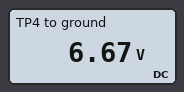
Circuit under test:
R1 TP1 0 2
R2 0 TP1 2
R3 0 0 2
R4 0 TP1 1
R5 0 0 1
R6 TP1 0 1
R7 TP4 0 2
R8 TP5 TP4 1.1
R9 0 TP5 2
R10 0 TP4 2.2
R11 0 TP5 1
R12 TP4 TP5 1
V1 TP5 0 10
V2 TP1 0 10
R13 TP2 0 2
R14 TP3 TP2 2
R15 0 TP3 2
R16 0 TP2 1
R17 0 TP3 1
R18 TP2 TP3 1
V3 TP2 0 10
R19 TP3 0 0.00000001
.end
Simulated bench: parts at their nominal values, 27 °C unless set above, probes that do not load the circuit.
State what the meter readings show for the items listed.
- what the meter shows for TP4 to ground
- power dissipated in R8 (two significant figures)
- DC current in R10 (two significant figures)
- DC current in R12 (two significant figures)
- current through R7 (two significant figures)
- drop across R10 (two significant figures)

6.67 V
10 W
3.0 A
3.3 A
3.3 A
6.7 V
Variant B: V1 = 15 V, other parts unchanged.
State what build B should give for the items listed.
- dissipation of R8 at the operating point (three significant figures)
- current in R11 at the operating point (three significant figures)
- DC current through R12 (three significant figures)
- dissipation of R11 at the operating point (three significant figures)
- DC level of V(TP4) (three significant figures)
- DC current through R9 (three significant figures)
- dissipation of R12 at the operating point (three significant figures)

22.7 W
15.0 A
5.00 A
225 W
10.0 V
7.50 A
25.0 W
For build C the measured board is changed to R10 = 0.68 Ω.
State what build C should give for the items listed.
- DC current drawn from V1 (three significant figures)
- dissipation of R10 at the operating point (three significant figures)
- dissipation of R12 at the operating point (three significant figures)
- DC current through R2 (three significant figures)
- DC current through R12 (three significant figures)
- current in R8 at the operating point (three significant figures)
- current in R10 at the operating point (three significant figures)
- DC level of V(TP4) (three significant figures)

24.7 A
35.6 W
25.8 W
5.00 A
5.08 A
4.62 A
7.24 A
4.92 V
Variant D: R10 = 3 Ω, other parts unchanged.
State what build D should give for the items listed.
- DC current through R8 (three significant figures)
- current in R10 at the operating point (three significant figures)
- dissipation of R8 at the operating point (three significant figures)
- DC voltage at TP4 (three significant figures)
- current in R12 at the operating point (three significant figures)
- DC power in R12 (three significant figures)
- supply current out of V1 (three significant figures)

2.76 A
2.32 A
8.39 W
6.96 V
3.04 A
9.23 W
20.8 A
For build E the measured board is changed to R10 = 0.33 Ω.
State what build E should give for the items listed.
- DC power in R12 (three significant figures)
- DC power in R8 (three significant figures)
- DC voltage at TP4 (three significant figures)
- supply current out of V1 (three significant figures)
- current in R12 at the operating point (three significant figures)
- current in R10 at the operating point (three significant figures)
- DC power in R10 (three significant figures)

42.1 W
38.3 W
3.51 V
27.4 A
6.49 A
10.6 A
37.3 W
